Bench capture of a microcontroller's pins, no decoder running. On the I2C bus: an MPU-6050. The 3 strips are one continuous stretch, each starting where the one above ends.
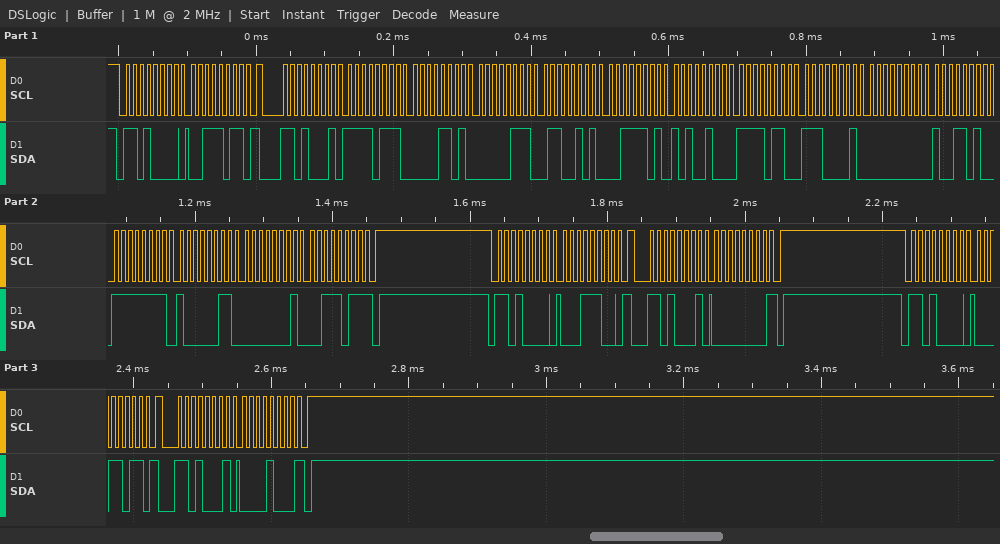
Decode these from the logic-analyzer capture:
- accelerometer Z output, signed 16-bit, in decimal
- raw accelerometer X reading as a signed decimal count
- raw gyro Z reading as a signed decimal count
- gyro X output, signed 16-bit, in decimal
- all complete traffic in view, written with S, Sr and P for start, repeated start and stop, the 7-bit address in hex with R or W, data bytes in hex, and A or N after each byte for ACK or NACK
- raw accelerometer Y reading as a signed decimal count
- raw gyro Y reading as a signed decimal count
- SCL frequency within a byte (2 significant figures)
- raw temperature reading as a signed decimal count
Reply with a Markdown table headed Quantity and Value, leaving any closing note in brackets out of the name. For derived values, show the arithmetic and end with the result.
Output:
| Quantity | Value |
|---|---|
| accelerometer Z output, signed 16-bit, in decimal | 0x3DA4 = 15780 |
| raw accelerometer X reading as a signed decimal count | 0xF70D = -2291 |
| raw gyro Z reading as a signed decimal count | 0x013B = 315 |
| gyro X output, signed 16-bit, in decimal | 0x009A = 154 |
| all complete traffic in view, written with S, Sr and P for start, repeated start and stop, the 7-bit address in hex with R or W, data bytes in hex, and A or N after each byte for ACK or NACK | S 68W A 3B A Sr 68R A F7 A 0D A 07 A 65 A 3D A A4 A F6 A E1 A 00 A 9A A FF A 83 A 01 A 3B N P S 68W A 1C A Sr 68R A 00 N P S 68W A 1B A Sr 68R A 08 N P |
| raw accelerometer Y reading as a signed decimal count | 0x0765 = 1893 |
| raw gyro Y reading as a signed decimal count | 0xFF83 = -125 |
| SCL frequency within a byte | 100 kHz |
| raw temperature reading as a signed decimal count | 0xF6E1 = -2335 |
